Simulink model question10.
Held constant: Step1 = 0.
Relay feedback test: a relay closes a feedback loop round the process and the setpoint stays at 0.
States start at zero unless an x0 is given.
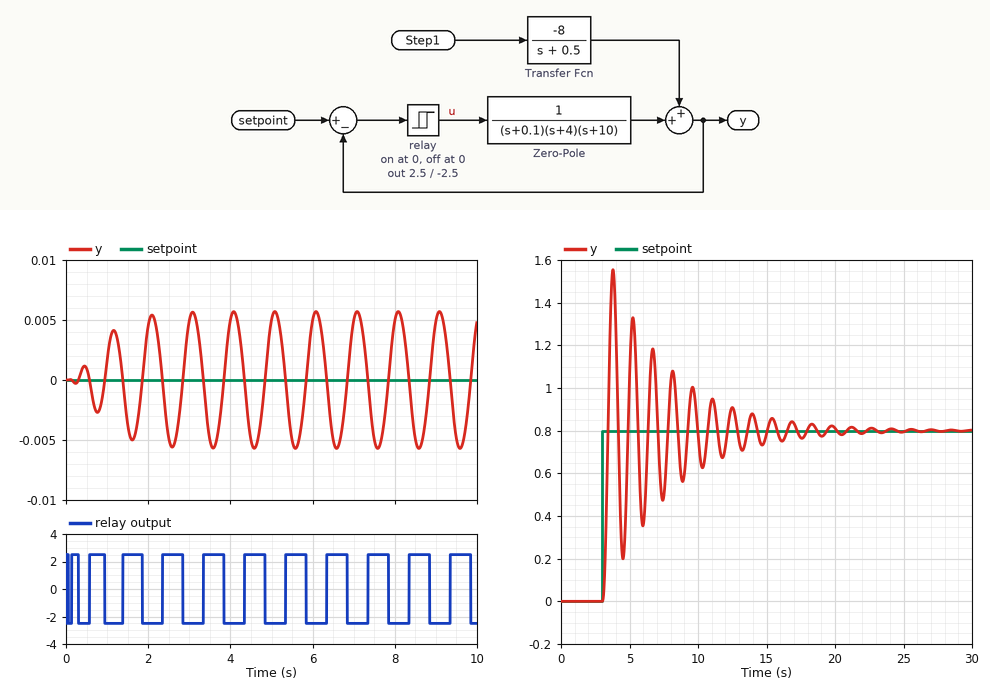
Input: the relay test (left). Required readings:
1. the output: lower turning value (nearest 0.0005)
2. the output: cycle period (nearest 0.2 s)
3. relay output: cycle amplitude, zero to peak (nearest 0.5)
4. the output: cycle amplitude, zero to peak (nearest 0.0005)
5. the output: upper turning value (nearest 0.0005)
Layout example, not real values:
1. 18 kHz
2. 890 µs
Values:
1. -0.0055
2. 1.0 s
3. 2.5
4. 0.0055
5. 0.0055
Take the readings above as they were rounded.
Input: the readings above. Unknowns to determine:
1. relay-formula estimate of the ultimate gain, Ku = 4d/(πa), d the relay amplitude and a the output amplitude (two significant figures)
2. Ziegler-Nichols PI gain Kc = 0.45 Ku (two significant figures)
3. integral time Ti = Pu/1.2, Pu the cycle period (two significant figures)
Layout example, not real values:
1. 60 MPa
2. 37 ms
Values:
1. 580
2. 260
3. 0.83 s
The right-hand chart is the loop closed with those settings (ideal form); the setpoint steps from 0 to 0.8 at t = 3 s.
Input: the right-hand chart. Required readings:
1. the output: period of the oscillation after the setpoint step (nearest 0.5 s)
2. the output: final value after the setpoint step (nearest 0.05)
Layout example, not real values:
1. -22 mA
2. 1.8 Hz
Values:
1. 1.5 s
2. 0.80
